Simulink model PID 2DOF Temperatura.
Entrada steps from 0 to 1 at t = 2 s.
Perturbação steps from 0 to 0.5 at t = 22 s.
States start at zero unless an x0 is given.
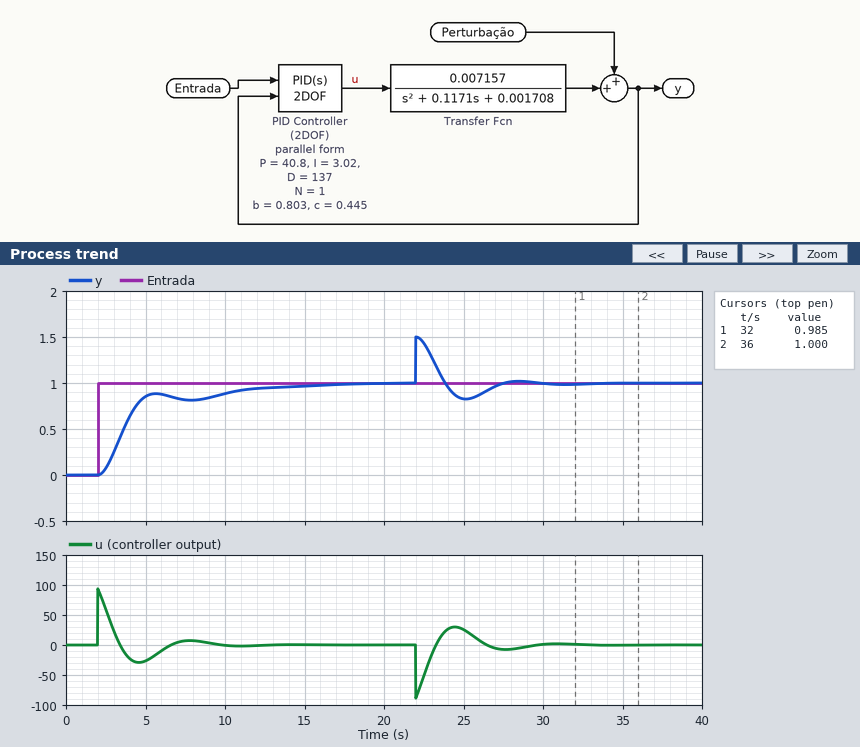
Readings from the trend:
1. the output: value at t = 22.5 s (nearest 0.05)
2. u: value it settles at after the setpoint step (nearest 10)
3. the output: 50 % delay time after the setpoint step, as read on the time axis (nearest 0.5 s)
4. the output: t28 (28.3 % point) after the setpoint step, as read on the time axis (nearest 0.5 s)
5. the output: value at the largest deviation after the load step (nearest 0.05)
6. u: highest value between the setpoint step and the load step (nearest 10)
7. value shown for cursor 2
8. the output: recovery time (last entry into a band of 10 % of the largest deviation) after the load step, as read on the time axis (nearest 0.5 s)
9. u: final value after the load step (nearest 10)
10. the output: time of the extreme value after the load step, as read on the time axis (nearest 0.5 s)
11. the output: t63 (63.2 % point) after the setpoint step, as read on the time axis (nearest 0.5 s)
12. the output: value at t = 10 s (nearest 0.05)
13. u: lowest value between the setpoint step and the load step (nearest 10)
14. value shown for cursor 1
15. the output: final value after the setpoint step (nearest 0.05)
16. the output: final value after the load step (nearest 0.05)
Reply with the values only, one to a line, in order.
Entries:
1.45
0
3.5 s
3.0 s
1.50
90
1.000
27.0 s
0
22.0 s
4.0 s
0.90
-30
0.985
1.00
1.00
